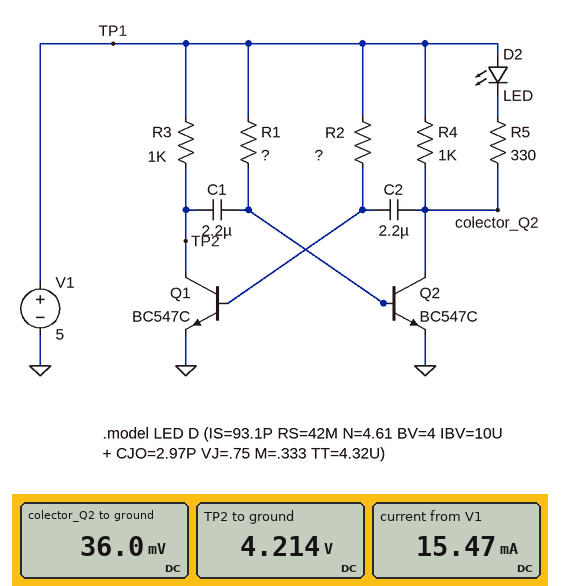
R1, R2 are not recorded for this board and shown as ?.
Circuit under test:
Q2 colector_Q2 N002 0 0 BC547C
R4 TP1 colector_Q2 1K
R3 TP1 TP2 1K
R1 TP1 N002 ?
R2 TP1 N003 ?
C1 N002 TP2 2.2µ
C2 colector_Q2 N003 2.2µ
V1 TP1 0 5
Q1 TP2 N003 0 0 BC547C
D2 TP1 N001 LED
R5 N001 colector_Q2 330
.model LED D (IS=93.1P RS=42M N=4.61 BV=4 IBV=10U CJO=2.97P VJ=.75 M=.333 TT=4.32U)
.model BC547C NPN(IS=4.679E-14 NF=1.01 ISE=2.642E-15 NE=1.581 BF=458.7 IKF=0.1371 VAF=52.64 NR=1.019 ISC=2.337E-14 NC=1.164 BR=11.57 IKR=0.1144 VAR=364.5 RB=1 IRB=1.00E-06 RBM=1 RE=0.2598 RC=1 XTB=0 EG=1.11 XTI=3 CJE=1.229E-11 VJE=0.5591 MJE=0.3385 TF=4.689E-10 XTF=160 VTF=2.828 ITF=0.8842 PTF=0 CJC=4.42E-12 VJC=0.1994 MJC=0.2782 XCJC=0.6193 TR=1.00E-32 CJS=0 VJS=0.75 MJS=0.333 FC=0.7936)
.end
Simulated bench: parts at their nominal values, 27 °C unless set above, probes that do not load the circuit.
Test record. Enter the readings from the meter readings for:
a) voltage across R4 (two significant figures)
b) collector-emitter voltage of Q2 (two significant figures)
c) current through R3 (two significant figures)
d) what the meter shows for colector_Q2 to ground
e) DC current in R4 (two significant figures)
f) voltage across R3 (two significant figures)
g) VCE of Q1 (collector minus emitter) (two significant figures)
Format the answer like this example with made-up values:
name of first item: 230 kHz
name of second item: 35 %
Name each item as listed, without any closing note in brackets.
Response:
voltage across R4: 5.0 V
collector-emitter voltage of Q2: 36 mV
current through R3: 790 µA
what the meter shows for colector_Q2 to ground: 36.0 mV
DC current in R4: 5.0 mA
voltage across R3: 790 mV
VCE of Q1 (collector minus emitter): 4.2 V
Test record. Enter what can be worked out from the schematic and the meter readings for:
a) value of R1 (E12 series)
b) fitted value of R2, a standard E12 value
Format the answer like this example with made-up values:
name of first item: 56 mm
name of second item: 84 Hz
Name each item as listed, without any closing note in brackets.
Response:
value of R1: 3.3 kΩ
fitted value of R2, a standard E12 value: 2.7 MΩ
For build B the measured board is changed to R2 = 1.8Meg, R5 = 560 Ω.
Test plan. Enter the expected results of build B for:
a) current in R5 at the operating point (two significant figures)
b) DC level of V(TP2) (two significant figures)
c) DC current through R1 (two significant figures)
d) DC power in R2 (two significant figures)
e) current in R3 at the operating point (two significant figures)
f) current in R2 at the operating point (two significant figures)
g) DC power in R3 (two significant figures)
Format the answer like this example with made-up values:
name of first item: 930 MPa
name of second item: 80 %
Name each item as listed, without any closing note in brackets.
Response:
current in R5 at the operating point: 5.1 mA
DC level of V(TP2): 3.8 V
DC current through R1: 1.3 mA
DC power in R2: 11 µW
current in R3 at the operating point: 1.2 mA
current in R2 at the operating point: 2.4 µA
DC power in R3: 1.4 mW
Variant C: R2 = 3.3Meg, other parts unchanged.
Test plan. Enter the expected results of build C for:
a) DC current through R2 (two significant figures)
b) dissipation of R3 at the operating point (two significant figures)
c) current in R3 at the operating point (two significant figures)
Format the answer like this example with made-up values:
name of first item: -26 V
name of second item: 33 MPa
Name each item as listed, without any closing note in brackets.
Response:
DC current through R2: 1.3 µA
dissipation of R3 at the operating point: 420 µW
current in R3 at the operating point: 650 µA
